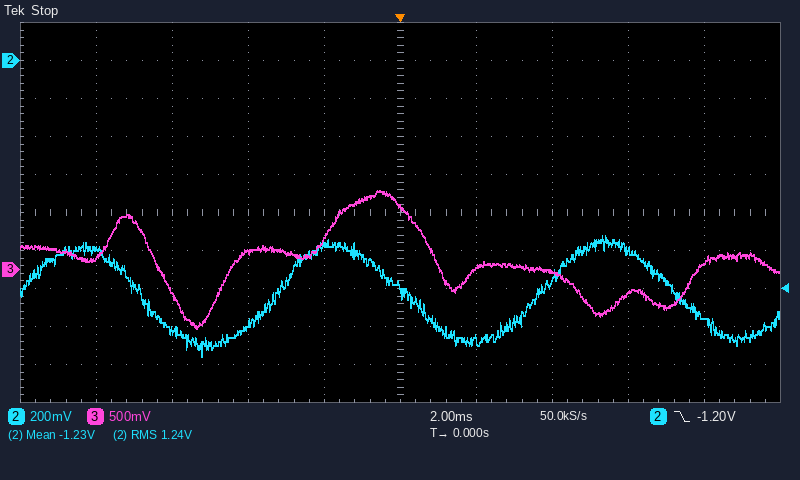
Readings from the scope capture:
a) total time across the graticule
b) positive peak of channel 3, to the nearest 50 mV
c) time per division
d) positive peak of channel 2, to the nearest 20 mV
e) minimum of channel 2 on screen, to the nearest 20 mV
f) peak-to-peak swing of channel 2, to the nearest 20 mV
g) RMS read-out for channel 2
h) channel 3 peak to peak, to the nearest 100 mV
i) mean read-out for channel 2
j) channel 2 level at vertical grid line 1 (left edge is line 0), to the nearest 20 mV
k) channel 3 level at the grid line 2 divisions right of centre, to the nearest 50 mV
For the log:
20 ms
1.05 V
2 ms
-920 mV
-1.56 V
640 mV
1.24 V
1.80 V
-1.23 V
-1.00 V
-50 mV
